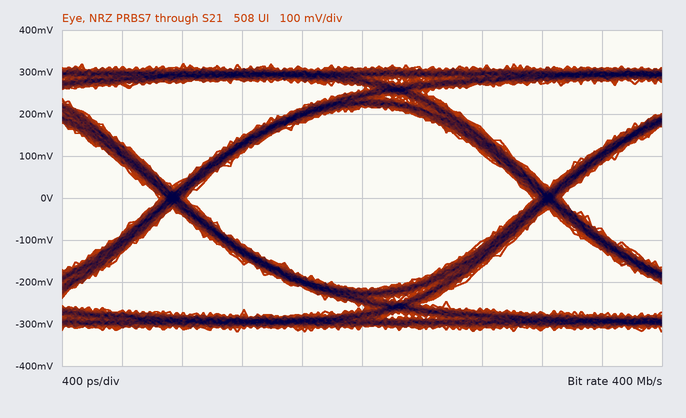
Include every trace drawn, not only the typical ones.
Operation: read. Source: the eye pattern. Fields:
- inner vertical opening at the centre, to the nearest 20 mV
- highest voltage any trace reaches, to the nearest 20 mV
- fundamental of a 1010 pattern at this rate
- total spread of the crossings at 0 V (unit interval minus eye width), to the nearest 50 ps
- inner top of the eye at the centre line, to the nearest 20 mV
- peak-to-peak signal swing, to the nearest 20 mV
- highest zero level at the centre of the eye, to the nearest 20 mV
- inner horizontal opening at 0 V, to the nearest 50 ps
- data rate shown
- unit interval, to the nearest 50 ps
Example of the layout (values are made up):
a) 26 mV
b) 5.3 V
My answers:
a) 440 mV
b) 320 mV
c) 200 MHz
d) 200 ps
e) 220 mV
f) 640 mV
g) -220 mV
h) 2.30 ns
i) 400 Mb/s
j) 2.50 ns
